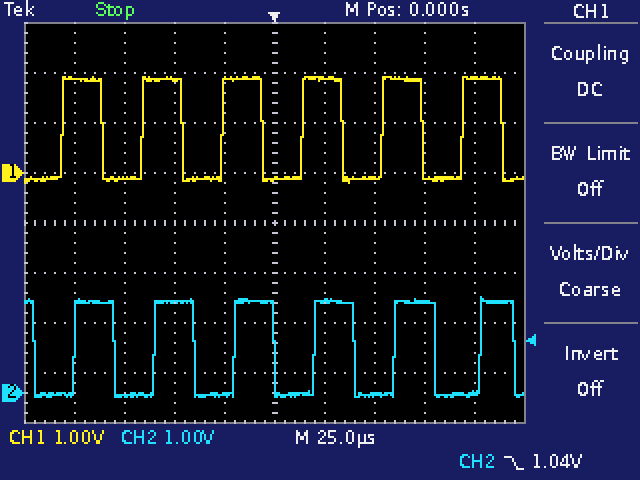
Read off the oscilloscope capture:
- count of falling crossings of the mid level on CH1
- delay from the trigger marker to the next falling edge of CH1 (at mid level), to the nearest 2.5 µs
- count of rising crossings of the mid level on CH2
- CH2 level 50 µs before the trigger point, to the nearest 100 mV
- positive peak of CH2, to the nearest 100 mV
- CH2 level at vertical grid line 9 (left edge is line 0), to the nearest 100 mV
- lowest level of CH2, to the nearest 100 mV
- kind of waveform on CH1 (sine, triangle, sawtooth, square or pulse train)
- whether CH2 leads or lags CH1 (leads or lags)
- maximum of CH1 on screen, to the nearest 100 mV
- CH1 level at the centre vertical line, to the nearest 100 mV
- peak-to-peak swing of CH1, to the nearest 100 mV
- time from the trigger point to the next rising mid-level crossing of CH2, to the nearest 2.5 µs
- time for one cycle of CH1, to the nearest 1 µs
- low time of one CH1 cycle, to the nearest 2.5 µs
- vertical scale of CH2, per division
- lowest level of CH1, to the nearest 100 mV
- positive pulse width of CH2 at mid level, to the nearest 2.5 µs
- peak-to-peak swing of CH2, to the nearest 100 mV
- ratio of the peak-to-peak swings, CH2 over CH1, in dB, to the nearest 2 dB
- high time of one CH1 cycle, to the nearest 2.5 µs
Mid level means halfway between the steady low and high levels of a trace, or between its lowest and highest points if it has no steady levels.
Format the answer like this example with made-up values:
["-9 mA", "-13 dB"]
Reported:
["6", "35.0 µs", "6", "1.8 V", "1.9 V", "0.0 V", "-100 mV", "square", "lags", "1.9 V", "-100 mV", "2.1 V", "20.0 µs", "40 µs", "20.0 µs", "1 V", "-200 mV", "20.0 µs", "2.0 V", "0 dB", "20.0 µs"]
